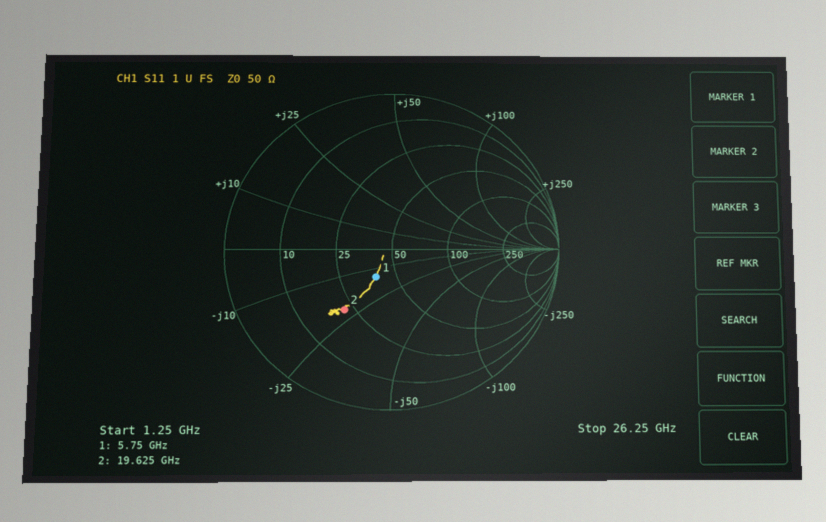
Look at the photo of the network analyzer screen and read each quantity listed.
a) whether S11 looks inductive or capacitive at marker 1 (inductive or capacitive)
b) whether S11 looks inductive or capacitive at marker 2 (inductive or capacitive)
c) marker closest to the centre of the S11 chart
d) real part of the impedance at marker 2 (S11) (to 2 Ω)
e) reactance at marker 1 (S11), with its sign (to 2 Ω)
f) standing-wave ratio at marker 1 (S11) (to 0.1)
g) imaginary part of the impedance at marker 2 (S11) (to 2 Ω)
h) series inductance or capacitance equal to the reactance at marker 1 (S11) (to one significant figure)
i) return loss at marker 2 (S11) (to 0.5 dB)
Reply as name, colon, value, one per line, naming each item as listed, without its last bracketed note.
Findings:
whether S11 looks inductive or capacitive at marker 1: capacitive
whether S11 looks inductive or capacitive at marker 2: capacitive
marker closest to the centre of the S11 chart: marker 1
real part of the impedance at marker 2 (S11): 22 Ω
reactance at marker 1 (S11), with its sign: -14 Ω
standing-wave ratio at marker 1 (S11): 1.5
imaginary part of the impedance at marker 2 (S11): -22 Ω
series inductance or capacitance equal to the reactance at marker 1 (S11): 2 pF
return loss at marker 2 (S11): 6.5 dB
